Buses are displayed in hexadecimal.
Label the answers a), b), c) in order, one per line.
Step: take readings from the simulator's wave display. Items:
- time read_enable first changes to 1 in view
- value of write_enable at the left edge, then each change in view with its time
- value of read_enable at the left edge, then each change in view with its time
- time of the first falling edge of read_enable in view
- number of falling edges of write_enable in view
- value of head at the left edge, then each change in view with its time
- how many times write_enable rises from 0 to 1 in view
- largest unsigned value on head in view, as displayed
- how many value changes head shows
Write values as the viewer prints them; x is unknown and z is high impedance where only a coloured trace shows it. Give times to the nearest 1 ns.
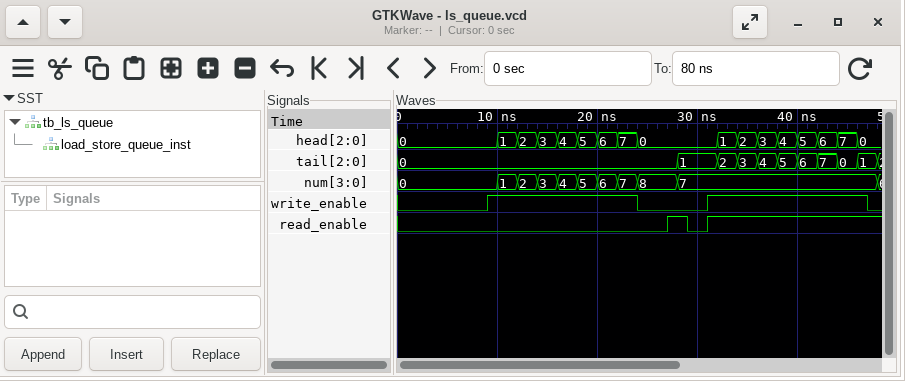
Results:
a) 27 ns
b) 0, 1 at 9 ns, 0 at 24 ns, 1 at 31 ns, 0 at 47 ns
c) 0, 1 at 27 ns, 0 at 29 ns, 1 at 31 ns
d) 29 ns
e) 2
f) 0, 1 at 10 ns, 2 at 12 ns, 3 at 14 ns, 4 at 16 ns, 5 at 18 ns, 6 at 20 ns, 7 at 22 ns, 0 at 24 ns, 1 at 32 ns, 2 at 34 ns, 3 at 36 ns, 4 at 38 ns, 5 at 40 ns, 6 at 42 ns, 7 at 44 ns, 0 at 46 ns
g) 2
h) 7
i) 16
